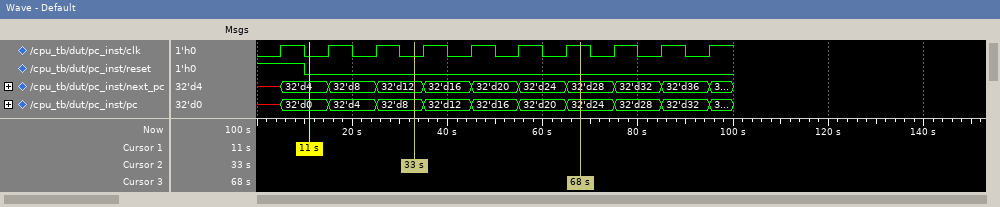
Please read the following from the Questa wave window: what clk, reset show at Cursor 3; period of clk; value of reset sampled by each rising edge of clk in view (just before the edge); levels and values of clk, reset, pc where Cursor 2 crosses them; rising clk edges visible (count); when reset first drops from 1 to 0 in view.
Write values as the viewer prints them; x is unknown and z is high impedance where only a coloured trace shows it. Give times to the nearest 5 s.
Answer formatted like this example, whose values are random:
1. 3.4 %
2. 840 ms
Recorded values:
1. clk=1, reset=0
2. 10 s
3. 1 0 0 0 0 0 0 0 0 0
4. clk=0, reset=0, pc=32'd8
5. 10
6. 10 s
